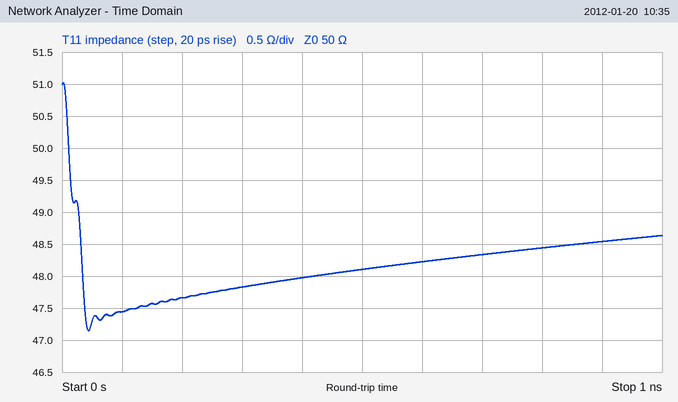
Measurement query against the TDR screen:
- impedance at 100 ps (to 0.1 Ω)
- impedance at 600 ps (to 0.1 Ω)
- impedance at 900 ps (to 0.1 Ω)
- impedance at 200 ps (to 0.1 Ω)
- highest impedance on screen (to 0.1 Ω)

47.4 Ω
48.2 Ω
48.5 Ω
47.7 Ω
51.0 Ω
